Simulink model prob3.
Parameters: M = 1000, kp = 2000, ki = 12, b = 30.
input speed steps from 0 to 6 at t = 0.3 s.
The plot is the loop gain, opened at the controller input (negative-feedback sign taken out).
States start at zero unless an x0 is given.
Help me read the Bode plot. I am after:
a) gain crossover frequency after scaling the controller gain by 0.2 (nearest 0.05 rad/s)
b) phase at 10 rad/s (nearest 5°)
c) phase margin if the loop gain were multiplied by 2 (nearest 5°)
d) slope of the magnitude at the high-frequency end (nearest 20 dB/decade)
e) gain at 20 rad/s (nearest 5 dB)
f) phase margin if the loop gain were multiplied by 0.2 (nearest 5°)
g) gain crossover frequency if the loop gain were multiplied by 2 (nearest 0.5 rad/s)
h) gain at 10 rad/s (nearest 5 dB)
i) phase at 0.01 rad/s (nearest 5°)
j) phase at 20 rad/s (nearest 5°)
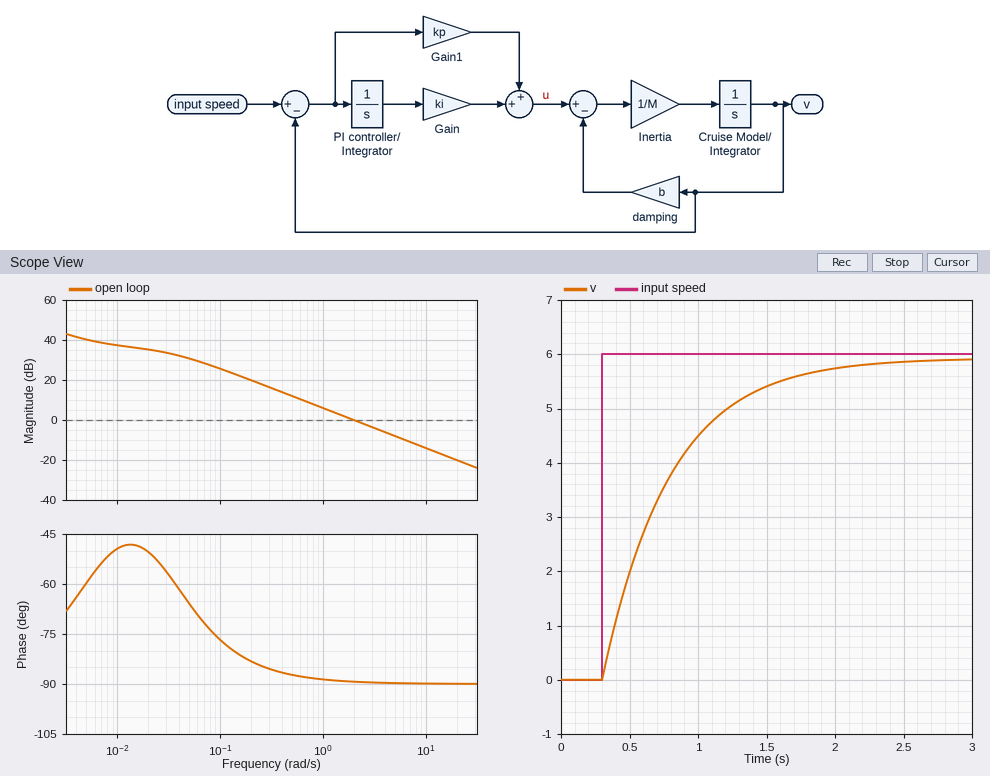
0.40 rad/s
-90°
90°
-20 dB/decade
-20 dB
95°
4.0 rad/s
-15 dB
-50°
-90°
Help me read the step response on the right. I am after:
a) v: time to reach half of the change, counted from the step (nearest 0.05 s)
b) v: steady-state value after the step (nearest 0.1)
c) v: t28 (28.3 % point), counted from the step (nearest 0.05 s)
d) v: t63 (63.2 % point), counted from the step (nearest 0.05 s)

0.35 s
5.9
0.15 s
0.50 s
